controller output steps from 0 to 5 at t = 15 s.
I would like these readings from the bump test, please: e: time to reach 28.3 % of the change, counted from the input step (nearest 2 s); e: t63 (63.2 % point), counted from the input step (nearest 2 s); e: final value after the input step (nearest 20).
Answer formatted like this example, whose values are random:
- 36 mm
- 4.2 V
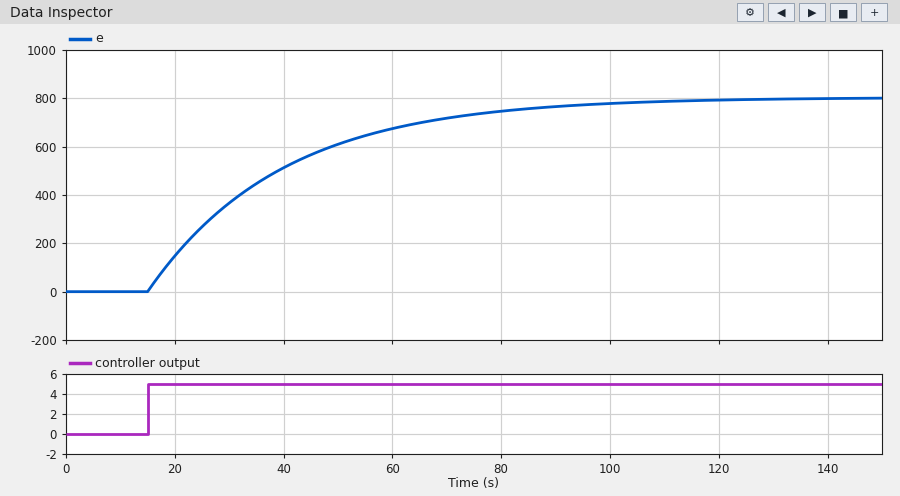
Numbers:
- 8 s
- 24 s
- 800
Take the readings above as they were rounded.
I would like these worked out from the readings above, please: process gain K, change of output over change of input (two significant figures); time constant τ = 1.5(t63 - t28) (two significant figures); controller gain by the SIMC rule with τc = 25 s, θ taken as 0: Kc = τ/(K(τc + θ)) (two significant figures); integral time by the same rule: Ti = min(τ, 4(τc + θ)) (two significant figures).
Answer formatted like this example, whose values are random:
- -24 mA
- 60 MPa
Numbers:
- 160
- 24 s
- 0.0060
- 24 s
